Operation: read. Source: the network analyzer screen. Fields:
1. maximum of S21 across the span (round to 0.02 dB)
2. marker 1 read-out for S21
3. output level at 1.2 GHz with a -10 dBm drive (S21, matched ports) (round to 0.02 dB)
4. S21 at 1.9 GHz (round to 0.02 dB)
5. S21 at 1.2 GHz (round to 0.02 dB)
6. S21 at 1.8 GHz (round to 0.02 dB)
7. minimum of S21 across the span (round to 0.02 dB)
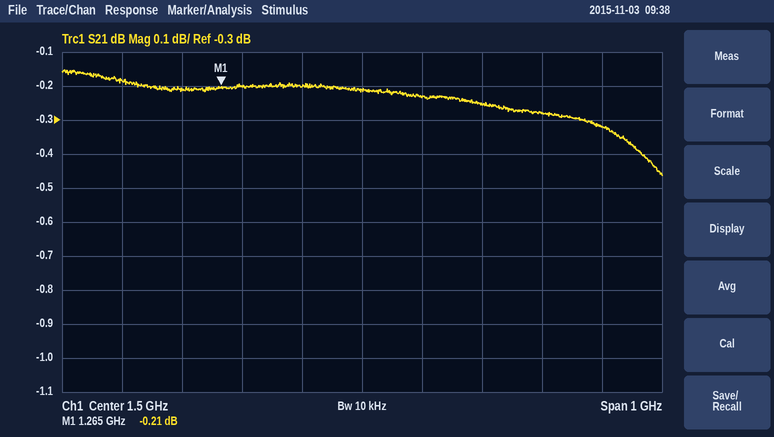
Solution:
-0.16 dB
-0.21 dB
-10.22 dBm
-0.32 dB
-0.22 dB
-0.28 dB
-0.46 dB
